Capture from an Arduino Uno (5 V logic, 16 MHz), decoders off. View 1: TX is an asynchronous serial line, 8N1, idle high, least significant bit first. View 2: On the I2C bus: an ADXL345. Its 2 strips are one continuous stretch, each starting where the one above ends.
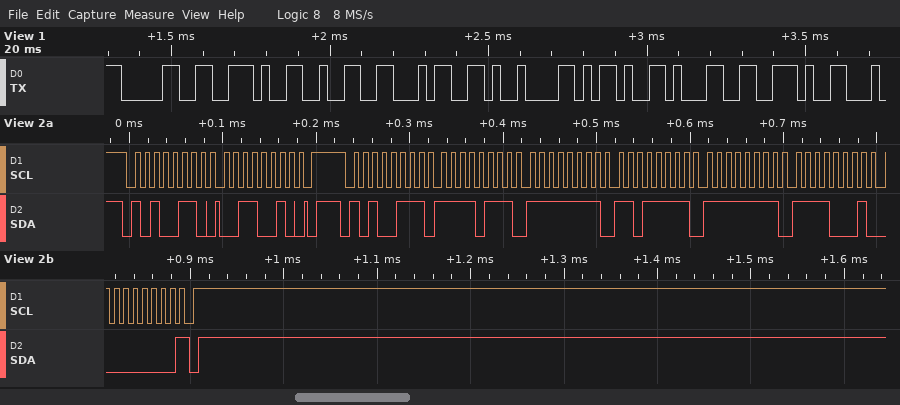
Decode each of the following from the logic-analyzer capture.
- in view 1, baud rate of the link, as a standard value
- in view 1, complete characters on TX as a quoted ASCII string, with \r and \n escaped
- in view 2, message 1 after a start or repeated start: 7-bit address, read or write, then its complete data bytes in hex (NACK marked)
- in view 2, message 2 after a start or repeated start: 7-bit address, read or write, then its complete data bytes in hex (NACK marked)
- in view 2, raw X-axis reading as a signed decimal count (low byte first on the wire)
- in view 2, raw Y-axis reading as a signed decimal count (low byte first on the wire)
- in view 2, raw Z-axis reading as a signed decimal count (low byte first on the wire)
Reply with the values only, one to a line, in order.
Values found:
38400 baud
"0.24\t-1."
0x53 write: 32
0x53 read: F7 FF DF FF F1 00 NACK
-9
-33
241
